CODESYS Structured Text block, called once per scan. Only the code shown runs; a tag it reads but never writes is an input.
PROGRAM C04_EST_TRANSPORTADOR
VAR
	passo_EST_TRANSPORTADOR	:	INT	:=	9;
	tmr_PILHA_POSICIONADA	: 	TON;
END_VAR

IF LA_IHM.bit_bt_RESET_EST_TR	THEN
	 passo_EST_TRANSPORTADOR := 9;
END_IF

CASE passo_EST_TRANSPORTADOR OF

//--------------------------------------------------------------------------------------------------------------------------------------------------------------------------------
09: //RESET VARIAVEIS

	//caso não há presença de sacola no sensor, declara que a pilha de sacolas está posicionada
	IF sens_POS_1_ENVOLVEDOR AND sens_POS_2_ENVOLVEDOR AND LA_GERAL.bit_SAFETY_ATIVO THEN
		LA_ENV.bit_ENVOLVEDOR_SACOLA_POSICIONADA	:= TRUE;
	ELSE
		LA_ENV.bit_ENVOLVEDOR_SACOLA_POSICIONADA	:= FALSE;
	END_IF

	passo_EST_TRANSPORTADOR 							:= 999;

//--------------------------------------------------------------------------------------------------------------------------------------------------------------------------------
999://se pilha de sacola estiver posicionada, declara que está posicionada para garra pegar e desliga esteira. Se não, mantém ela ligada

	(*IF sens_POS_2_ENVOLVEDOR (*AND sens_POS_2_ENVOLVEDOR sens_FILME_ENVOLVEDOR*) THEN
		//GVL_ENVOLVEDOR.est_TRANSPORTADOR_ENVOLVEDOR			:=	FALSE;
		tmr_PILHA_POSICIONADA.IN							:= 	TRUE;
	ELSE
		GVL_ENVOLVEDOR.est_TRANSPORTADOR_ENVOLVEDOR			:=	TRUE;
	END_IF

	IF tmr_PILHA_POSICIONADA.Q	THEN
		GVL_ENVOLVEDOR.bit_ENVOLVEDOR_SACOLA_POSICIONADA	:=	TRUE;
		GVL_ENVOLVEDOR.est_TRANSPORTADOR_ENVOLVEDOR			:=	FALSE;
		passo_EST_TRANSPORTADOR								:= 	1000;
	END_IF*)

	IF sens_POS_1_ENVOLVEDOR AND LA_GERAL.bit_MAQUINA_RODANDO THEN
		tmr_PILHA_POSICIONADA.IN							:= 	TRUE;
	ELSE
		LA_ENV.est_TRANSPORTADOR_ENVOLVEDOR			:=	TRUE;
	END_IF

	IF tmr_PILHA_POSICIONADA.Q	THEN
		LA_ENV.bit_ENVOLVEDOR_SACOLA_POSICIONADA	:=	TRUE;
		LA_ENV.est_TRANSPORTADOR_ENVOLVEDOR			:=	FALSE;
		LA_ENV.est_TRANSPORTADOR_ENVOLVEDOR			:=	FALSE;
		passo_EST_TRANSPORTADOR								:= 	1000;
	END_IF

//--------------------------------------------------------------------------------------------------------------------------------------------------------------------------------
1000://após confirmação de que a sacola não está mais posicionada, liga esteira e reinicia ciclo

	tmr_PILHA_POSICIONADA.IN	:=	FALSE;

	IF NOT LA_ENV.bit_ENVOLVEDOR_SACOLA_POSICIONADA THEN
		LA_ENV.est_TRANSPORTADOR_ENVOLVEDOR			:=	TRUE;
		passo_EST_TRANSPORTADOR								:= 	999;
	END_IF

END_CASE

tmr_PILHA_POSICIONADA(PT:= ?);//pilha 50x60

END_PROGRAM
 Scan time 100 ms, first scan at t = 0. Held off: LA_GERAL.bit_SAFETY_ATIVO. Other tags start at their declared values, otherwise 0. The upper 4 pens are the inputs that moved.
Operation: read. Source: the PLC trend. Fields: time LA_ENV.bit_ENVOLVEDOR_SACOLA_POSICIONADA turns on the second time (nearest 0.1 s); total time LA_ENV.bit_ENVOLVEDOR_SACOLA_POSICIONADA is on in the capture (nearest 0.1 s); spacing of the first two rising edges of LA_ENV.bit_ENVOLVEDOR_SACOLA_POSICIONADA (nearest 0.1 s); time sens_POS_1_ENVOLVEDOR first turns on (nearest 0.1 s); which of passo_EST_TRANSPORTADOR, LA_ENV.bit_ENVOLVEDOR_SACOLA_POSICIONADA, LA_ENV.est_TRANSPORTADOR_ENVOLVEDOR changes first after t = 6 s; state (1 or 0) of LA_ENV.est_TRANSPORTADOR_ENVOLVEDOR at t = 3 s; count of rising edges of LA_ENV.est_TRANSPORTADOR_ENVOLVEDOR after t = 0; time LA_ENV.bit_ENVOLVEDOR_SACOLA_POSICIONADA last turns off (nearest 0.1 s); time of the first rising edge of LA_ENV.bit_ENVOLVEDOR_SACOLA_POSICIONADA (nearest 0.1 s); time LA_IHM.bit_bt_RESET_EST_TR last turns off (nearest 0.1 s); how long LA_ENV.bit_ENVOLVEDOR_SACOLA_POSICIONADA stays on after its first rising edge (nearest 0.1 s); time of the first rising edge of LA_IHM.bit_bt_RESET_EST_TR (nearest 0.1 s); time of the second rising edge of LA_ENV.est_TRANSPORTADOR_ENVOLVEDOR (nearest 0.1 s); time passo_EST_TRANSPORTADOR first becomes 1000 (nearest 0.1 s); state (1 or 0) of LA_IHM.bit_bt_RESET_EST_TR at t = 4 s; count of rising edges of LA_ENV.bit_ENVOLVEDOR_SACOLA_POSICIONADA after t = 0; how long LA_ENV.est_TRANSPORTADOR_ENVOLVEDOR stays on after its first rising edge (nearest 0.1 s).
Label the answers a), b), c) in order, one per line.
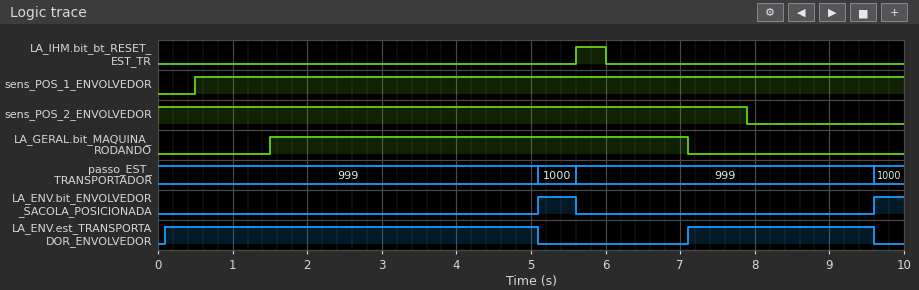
a) 9.6 s
b) 0.9 s
c) 4.5 s
d) 0.5 s
e) LA_ENV.est_TRANSPORTADOR_ENVOLVEDOR
f) 1
g) 2
h) 5.6 s
i) 5.1 s
j) 6.0 s
k) 0.5 s
l) 5.6 s
m) 7.1 s
n) 5.1 s
o) 0
p) 2
q) 5.0 s
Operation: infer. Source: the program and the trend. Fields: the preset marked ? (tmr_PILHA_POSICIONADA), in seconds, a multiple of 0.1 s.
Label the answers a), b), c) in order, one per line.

a) 3.5 s
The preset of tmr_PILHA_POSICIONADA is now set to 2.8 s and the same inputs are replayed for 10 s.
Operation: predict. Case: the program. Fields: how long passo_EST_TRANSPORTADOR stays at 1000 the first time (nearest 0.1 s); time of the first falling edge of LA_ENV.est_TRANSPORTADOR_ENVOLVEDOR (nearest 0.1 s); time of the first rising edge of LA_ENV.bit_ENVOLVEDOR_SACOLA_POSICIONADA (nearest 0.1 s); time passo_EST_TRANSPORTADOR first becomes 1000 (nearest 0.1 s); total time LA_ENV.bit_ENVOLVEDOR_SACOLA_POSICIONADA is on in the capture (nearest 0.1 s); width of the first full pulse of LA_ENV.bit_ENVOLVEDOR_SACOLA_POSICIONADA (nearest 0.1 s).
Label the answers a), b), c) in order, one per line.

a) 1.2 s
b) 4.4 s
c) 4.4 s
d) 4.4 s
e) 2.3 s
f) 1.2 s
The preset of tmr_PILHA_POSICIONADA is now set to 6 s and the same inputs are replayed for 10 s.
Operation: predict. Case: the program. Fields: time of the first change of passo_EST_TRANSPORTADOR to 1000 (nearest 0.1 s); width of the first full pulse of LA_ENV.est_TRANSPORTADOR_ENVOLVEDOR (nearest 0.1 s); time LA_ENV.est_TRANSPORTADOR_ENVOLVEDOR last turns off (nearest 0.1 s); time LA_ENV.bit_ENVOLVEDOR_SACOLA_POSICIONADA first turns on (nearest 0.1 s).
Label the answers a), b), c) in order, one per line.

a) 7.6 s
b) 7.5 s
c) 7.6 s
d) 7.6 s
